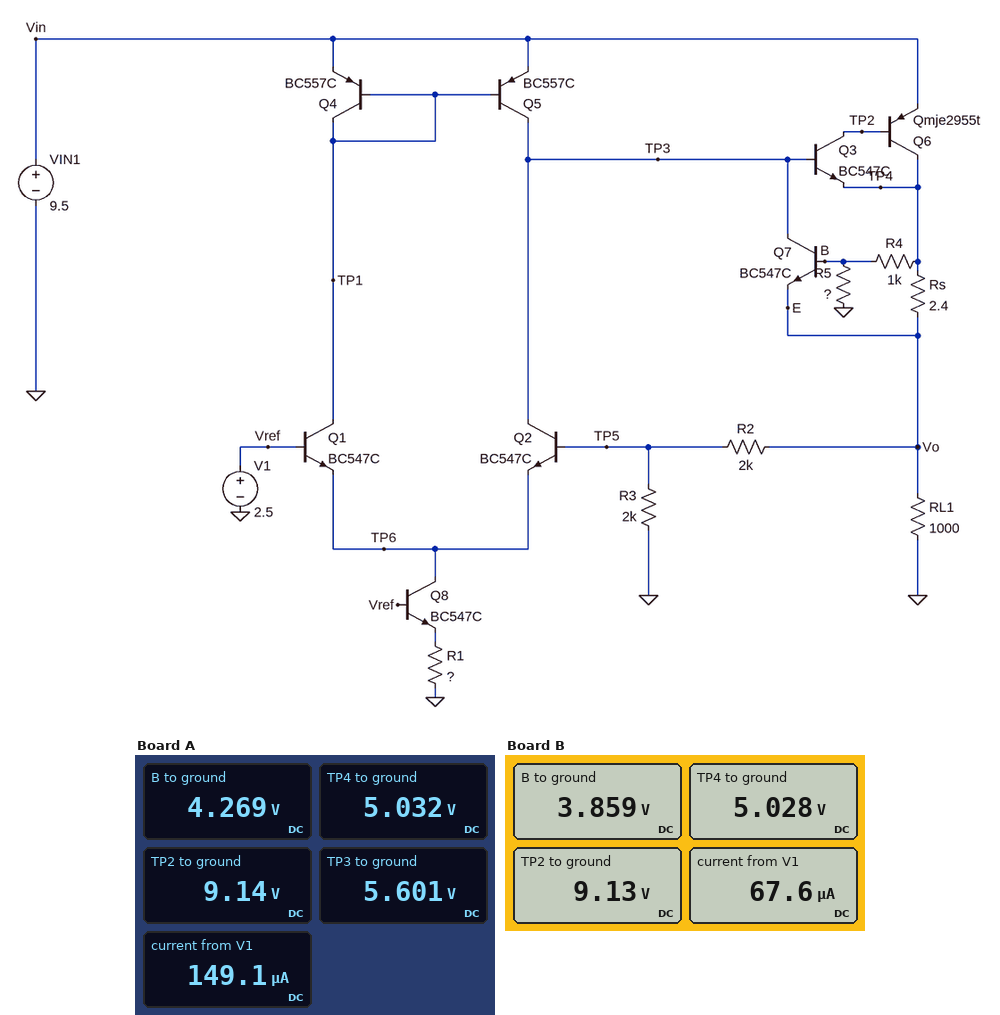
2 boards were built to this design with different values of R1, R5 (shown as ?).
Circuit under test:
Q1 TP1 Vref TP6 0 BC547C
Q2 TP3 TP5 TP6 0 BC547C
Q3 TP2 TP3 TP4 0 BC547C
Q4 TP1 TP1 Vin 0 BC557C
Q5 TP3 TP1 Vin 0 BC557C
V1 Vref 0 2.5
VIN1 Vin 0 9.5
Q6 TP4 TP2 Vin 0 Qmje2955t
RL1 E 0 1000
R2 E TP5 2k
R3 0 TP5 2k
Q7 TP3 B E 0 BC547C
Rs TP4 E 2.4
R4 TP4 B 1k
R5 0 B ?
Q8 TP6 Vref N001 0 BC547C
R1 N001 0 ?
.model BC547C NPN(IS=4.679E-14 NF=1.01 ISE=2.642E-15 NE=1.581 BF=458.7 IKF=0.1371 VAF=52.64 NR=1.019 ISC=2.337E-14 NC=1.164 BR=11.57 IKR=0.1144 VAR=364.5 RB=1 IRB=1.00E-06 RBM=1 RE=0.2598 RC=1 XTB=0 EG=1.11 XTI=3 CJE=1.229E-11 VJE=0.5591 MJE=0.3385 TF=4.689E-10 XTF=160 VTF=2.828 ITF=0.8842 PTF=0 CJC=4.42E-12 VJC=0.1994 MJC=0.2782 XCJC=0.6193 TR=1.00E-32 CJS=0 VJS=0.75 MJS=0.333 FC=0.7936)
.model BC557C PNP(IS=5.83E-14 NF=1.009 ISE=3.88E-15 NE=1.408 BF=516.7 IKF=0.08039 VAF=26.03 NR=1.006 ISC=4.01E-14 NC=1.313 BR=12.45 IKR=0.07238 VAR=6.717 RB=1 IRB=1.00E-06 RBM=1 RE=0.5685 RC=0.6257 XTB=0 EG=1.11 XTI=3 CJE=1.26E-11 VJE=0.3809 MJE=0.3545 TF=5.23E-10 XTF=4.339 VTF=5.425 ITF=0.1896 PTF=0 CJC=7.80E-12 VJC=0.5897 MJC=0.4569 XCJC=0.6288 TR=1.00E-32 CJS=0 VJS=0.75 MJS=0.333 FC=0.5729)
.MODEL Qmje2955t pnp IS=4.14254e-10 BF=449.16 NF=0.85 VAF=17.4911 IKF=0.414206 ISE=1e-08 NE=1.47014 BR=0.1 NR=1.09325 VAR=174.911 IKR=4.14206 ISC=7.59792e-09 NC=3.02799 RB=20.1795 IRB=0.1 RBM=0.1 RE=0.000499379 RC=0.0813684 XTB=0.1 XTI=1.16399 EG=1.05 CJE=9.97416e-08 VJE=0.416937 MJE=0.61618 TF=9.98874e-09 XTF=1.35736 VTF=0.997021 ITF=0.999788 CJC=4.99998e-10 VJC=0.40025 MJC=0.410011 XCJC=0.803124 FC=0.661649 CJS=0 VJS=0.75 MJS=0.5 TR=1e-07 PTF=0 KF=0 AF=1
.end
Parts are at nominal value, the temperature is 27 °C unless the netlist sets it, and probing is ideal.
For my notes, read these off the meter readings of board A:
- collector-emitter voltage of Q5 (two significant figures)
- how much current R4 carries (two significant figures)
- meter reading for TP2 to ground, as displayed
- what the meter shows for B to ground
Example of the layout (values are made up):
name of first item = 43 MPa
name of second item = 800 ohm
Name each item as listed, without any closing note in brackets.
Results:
collector-emitter voltage of Q5 = -3.9 V
how much current R4 carries = 760 µA
meter reading for TP2 to ground, as displayed = 9.14 V
what the meter shows for B to ground = 4.269 V
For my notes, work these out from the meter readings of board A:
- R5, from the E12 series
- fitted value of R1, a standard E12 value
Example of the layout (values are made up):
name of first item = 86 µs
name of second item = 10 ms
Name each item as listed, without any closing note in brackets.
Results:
R5, from the E12 series = 5.6 kΩ
fitted value of R1, a standard E12 value = 560 Ω
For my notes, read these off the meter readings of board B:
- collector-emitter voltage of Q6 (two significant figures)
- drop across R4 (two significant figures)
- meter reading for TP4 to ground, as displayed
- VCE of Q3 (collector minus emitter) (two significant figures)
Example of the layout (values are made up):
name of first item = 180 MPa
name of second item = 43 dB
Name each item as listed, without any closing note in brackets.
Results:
collector-emitter voltage of Q6 = -4.5 V
drop across R4 = 1.2 V
meter reading for TP4 to ground, as displayed = 5.028 V
VCE of Q3 (collector minus emitter) = 4.1 V
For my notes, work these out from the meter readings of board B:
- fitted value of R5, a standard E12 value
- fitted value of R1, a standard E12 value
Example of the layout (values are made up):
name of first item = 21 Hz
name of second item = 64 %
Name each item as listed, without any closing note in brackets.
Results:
fitted value of R5, a standard E12 value = 3.3 kΩ
fitted value of R1, a standard E12 value = 1.2 kΩ
